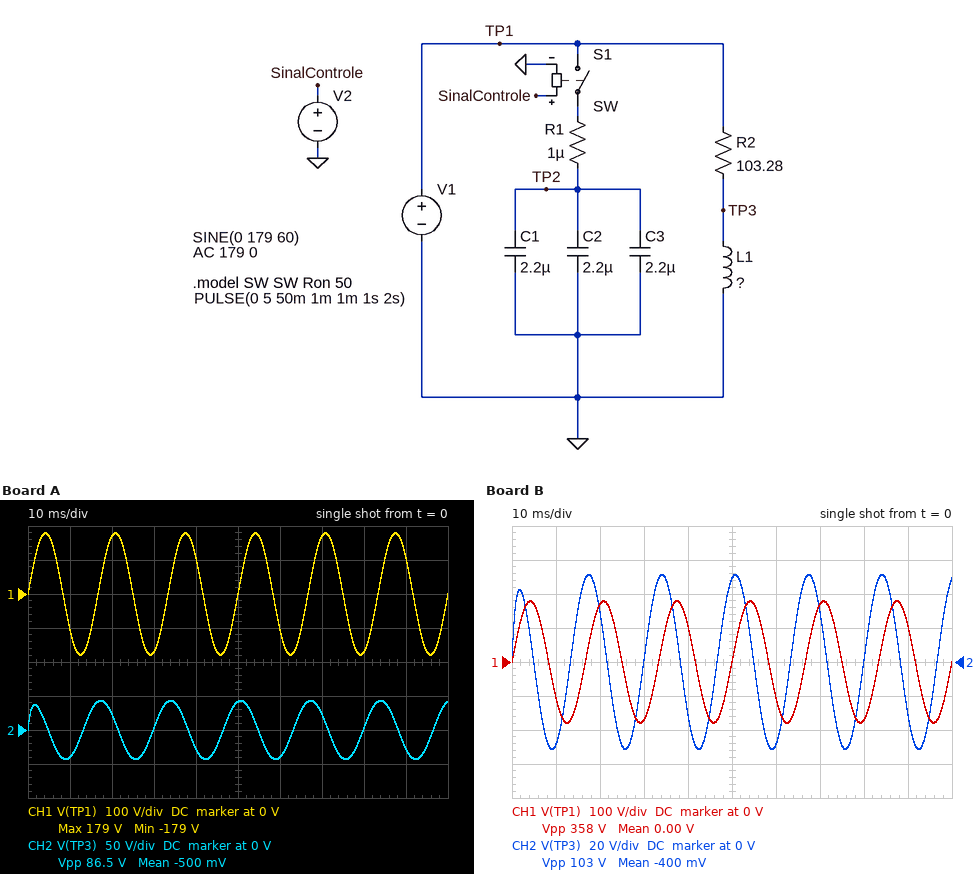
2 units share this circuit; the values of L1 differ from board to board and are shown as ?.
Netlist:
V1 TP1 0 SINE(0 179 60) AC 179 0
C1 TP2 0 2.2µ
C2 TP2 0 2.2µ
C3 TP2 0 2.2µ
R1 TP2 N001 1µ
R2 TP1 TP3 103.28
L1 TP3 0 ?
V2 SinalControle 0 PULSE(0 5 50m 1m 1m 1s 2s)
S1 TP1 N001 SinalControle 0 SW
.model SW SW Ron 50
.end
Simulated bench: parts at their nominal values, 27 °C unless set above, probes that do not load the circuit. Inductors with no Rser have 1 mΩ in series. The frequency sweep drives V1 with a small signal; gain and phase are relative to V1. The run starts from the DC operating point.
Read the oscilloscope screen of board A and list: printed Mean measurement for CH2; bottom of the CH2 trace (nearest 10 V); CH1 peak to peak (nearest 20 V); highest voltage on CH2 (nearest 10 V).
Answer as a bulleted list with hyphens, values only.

- -500 mV
- -40 V
- 360 V
- 40 V
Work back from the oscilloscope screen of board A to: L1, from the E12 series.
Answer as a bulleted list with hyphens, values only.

- 68 mH
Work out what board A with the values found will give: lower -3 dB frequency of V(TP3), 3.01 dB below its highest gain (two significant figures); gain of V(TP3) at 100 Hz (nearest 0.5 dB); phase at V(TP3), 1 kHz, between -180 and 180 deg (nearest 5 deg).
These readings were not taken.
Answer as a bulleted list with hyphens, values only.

- 240 Hz
- -8.5 dB
- 15 deg
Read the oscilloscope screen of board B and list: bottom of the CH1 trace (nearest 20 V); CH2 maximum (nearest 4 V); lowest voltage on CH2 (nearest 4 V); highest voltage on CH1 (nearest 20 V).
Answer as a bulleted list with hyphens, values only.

- -180 V
- 52 V
- -52 V
- 180 V
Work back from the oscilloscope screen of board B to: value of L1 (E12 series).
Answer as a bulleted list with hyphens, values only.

- 82 mH
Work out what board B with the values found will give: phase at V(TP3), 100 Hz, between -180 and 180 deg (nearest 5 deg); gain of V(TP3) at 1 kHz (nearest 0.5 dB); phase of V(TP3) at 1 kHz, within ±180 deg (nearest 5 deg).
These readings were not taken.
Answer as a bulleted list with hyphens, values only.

- 65 deg
- 0 dB
- 10 deg
